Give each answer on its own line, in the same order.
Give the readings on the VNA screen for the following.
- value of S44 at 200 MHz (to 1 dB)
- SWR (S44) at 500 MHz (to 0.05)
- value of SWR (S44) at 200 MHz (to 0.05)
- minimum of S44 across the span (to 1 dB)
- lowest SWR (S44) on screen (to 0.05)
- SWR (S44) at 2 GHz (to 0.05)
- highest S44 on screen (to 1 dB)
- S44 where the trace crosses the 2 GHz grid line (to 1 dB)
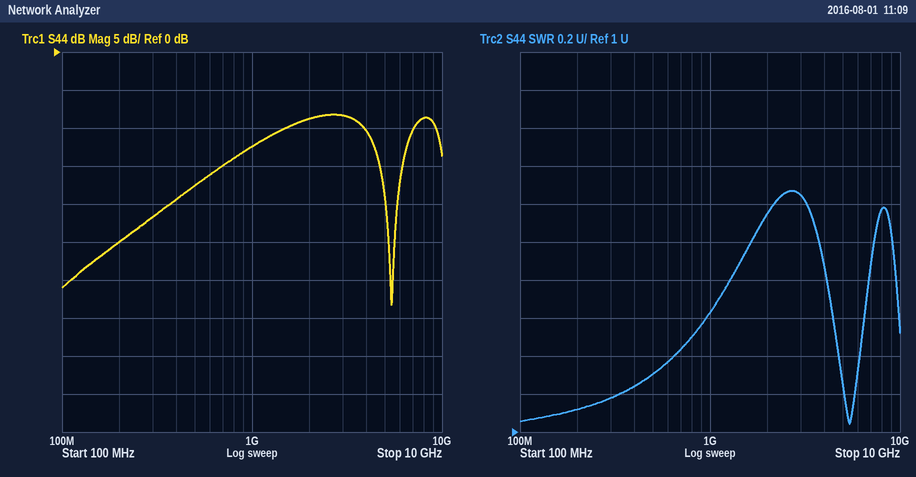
-25 dB
1.30
1.10
-33 dB
1.05
2.15
-8 dB
-9 dB
